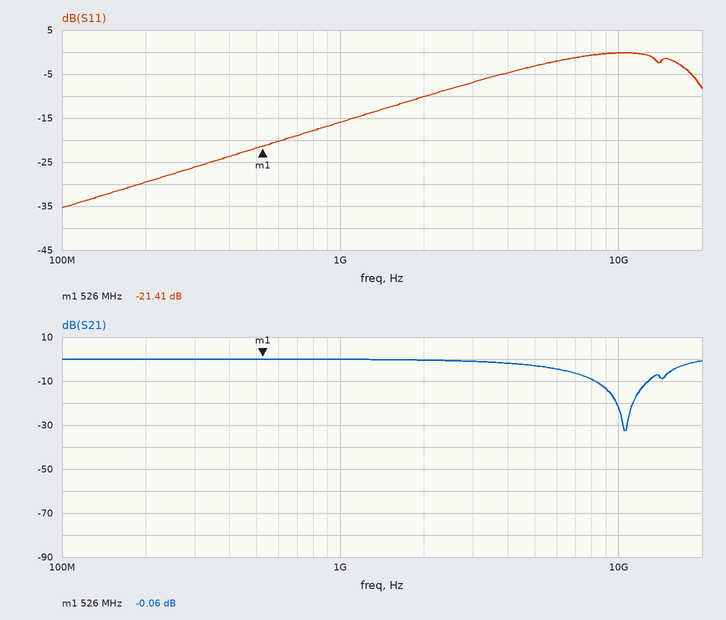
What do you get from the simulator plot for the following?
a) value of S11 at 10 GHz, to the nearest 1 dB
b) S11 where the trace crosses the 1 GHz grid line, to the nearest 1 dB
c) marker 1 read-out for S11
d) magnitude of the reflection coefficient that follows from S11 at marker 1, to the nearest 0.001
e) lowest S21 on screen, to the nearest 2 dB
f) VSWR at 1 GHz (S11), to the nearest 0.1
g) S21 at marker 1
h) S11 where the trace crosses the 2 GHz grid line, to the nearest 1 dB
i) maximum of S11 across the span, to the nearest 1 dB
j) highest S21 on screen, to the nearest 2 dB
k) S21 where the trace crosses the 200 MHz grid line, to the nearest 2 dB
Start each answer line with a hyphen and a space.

- 0 dB
- -16 dB
- -21.41 dB
- 0.085
- -32 dB
- 1.4
- -0.06 dB
- -10 dB
- 0 dB
- 0 dB
- 0 dB
